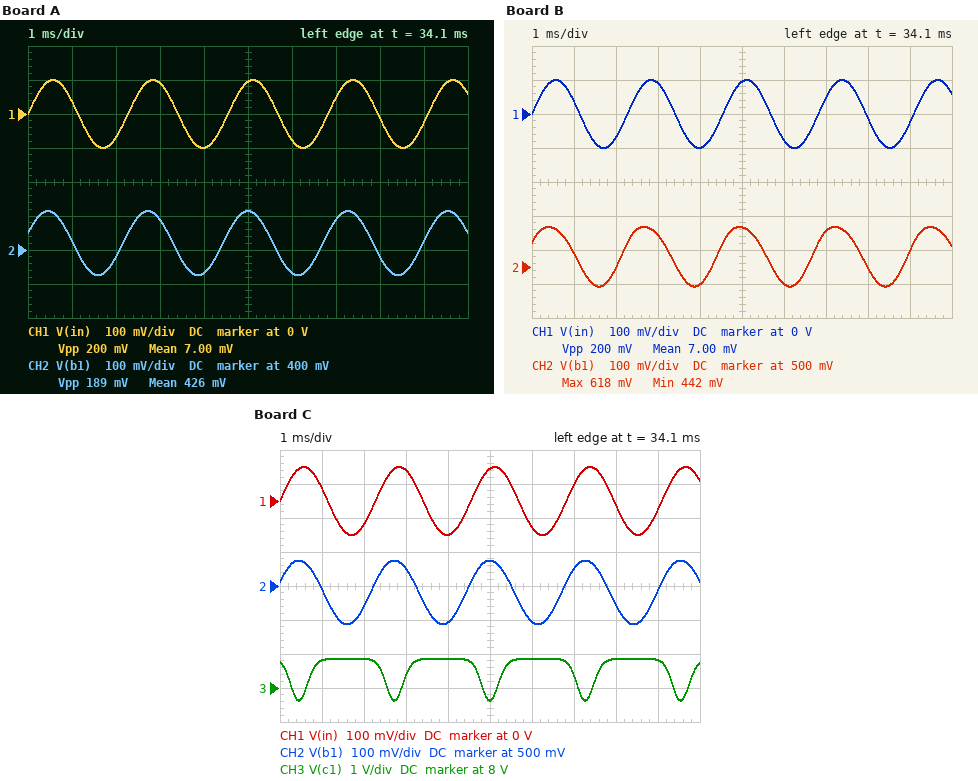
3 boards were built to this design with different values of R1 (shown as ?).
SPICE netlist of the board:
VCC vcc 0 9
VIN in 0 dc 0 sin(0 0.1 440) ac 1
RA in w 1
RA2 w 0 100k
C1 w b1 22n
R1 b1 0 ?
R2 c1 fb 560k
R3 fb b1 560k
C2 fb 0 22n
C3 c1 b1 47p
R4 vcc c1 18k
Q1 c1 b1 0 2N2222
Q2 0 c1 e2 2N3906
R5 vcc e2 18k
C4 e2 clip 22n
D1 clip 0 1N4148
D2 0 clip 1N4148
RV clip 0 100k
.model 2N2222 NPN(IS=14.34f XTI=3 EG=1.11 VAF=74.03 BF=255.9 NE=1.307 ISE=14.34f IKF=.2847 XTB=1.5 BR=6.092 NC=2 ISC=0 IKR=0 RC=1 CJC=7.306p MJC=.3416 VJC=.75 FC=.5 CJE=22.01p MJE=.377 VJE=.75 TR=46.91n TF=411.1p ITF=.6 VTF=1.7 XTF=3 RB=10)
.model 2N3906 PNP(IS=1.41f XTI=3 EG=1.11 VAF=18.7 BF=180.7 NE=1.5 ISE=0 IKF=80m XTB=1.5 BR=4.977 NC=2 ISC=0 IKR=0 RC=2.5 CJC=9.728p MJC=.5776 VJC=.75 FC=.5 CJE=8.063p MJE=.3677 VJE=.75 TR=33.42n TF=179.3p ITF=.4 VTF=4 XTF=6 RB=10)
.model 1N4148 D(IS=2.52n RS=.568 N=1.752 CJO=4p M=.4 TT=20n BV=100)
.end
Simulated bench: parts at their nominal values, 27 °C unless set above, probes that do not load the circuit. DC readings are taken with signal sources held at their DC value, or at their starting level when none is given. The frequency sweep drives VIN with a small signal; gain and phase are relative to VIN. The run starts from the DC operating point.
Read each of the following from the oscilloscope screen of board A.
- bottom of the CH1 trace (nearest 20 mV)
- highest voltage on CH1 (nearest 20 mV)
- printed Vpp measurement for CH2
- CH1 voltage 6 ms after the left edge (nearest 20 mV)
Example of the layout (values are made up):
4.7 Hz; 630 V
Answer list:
-100 mV; 100 mV; 189 mV; -80 mV
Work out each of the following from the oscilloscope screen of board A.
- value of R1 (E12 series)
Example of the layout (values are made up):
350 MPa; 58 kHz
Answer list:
56 kΩ
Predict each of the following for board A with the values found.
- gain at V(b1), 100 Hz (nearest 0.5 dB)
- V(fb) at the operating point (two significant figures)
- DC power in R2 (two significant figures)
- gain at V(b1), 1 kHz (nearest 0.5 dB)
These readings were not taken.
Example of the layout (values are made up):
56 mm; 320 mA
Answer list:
-5.0 dB; 4.6 V; 32 µW; 0 dB
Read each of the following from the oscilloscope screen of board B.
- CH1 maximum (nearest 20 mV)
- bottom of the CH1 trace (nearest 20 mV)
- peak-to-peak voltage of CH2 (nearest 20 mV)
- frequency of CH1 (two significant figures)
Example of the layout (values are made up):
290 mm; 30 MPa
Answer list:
100 mV; -100 mV; 180 mV; 440 Hz
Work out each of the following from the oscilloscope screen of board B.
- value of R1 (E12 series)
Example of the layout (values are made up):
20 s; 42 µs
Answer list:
100 kΩ
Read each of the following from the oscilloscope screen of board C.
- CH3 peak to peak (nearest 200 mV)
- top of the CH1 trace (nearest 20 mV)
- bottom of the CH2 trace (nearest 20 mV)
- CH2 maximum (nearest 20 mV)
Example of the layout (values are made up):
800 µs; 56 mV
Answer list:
1.2 V; 100 mV; 380 mV; 580 mV
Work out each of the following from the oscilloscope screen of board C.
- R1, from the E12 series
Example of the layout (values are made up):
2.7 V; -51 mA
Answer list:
68 kΩ
